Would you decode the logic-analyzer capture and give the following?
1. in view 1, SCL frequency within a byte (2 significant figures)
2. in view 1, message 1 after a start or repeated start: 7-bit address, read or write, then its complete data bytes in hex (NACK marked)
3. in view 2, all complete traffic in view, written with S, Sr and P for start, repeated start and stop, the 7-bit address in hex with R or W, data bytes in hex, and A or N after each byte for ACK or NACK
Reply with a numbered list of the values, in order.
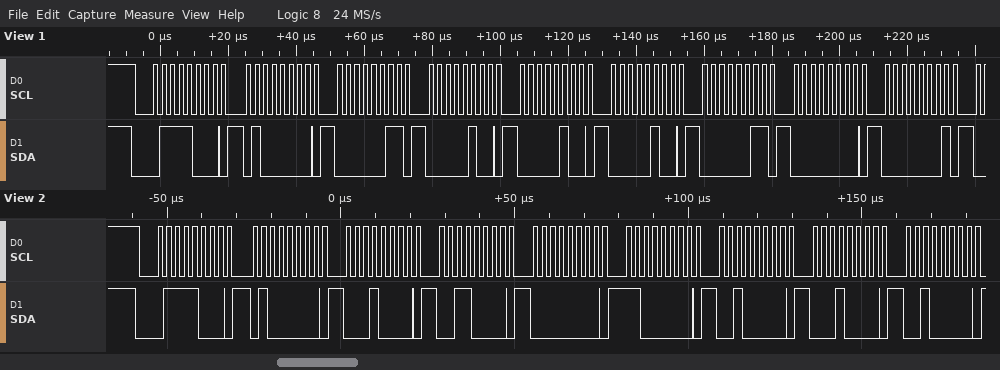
1. 400 kHz
2. 0x3C write: 40 03 04 04 04 03 00 01
3. S 3CW A 40 A 10 A 30 A 00 A C0 A 20 A 10 A 20 A
